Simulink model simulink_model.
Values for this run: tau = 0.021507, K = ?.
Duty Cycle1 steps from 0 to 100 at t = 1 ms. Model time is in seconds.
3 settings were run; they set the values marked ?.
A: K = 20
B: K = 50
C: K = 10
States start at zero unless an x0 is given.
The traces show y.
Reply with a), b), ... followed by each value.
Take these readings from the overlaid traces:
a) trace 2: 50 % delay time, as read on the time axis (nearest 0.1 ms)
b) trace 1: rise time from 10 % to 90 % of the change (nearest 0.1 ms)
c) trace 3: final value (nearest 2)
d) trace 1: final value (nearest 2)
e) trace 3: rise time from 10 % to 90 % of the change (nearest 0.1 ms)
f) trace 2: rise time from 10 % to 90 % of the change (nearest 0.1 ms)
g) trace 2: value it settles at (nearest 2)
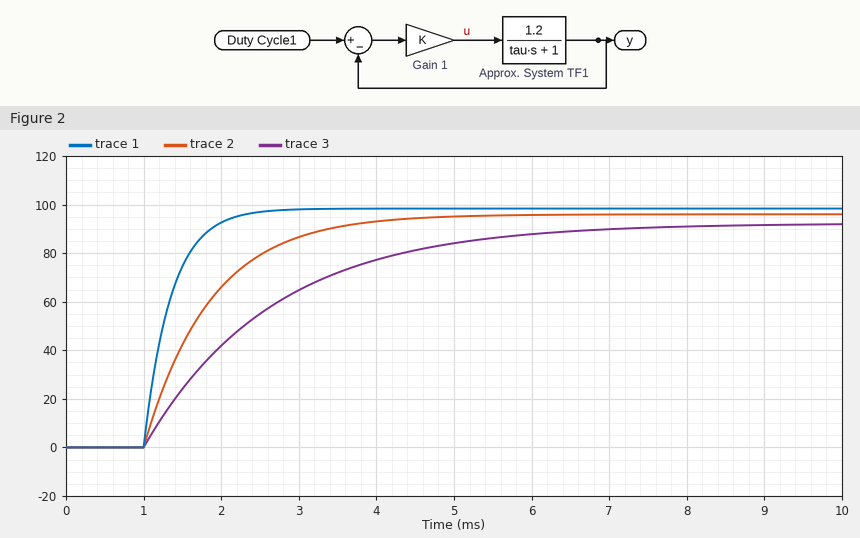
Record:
a) 1.6 ms
b) 0.8 ms
c) 92
d) 98
e) 3.6 ms
f) 1.9 ms
g) 96
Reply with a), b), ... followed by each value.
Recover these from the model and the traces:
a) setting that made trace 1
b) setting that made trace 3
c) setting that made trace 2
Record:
a) B
b) C
c) A
